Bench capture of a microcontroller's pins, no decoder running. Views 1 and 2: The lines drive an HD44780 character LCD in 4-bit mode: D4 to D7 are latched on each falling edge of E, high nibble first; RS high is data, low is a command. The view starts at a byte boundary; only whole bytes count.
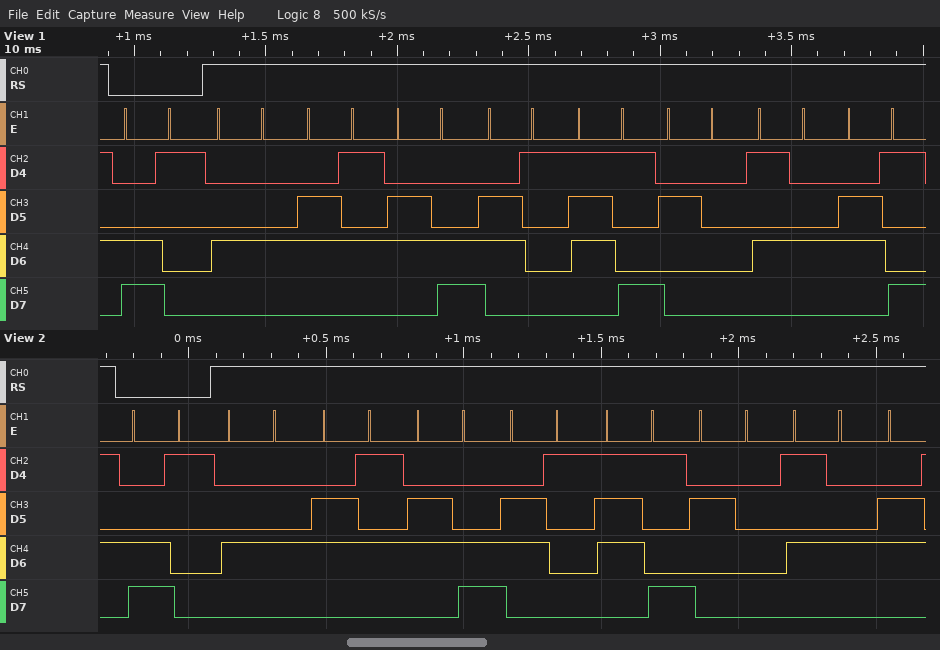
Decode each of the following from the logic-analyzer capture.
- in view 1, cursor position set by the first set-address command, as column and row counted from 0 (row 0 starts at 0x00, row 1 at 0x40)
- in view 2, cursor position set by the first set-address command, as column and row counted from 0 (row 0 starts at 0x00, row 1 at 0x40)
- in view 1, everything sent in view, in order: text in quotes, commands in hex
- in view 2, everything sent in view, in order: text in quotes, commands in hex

column 1, row 1
column 1, row 1
0xC1 "Delay Ti"
0xC1 "Delay T"
